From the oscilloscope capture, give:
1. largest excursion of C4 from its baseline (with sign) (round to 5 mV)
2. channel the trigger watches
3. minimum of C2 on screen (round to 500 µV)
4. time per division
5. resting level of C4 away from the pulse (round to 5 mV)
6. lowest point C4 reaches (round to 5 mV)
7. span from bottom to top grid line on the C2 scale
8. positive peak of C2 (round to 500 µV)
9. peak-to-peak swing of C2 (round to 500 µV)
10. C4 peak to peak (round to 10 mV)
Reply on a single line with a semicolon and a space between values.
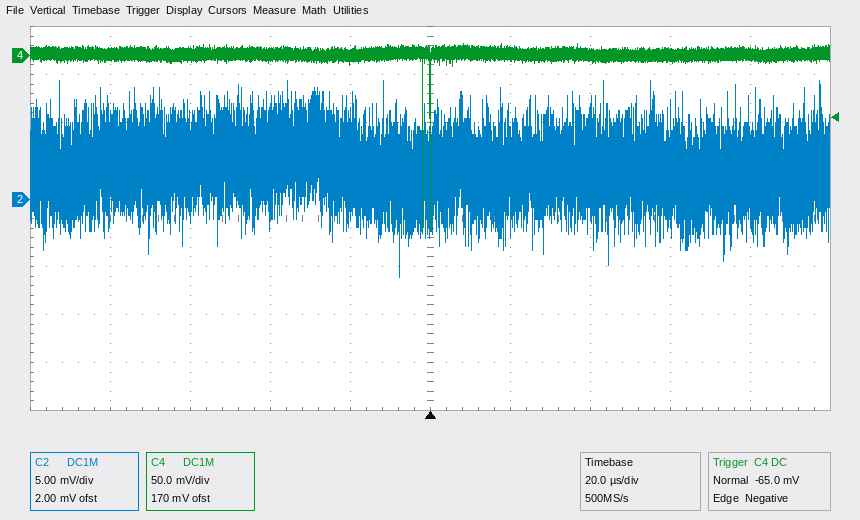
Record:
-185 mV; C4; -8.0 mV; 20 µs; 0 mV; -185 mV; 40 mV; 12.5 mV; 20.5 mV; 200 mV
